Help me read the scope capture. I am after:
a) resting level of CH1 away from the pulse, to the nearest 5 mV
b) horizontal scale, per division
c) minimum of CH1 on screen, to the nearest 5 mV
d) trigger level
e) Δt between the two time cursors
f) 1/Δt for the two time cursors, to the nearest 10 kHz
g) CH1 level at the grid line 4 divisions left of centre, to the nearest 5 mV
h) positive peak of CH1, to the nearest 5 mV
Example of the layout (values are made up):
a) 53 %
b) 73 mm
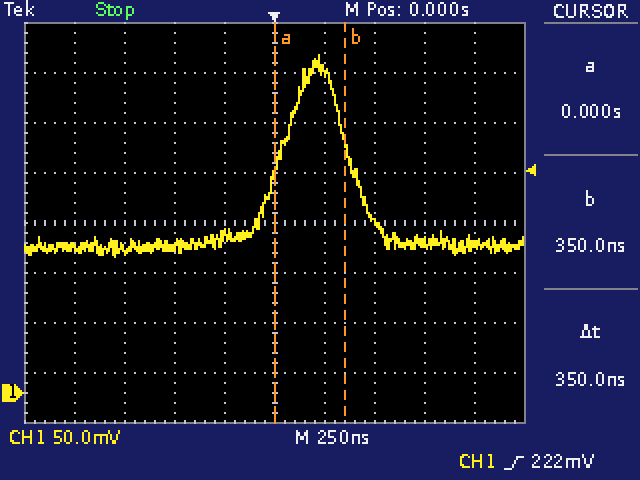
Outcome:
a) 145 mV
b) 250 ns
c) 135 mV
d) 222 mV
e) 350 ns
f) 2.86 MHz
g) 145 mV
h) 340 mV
